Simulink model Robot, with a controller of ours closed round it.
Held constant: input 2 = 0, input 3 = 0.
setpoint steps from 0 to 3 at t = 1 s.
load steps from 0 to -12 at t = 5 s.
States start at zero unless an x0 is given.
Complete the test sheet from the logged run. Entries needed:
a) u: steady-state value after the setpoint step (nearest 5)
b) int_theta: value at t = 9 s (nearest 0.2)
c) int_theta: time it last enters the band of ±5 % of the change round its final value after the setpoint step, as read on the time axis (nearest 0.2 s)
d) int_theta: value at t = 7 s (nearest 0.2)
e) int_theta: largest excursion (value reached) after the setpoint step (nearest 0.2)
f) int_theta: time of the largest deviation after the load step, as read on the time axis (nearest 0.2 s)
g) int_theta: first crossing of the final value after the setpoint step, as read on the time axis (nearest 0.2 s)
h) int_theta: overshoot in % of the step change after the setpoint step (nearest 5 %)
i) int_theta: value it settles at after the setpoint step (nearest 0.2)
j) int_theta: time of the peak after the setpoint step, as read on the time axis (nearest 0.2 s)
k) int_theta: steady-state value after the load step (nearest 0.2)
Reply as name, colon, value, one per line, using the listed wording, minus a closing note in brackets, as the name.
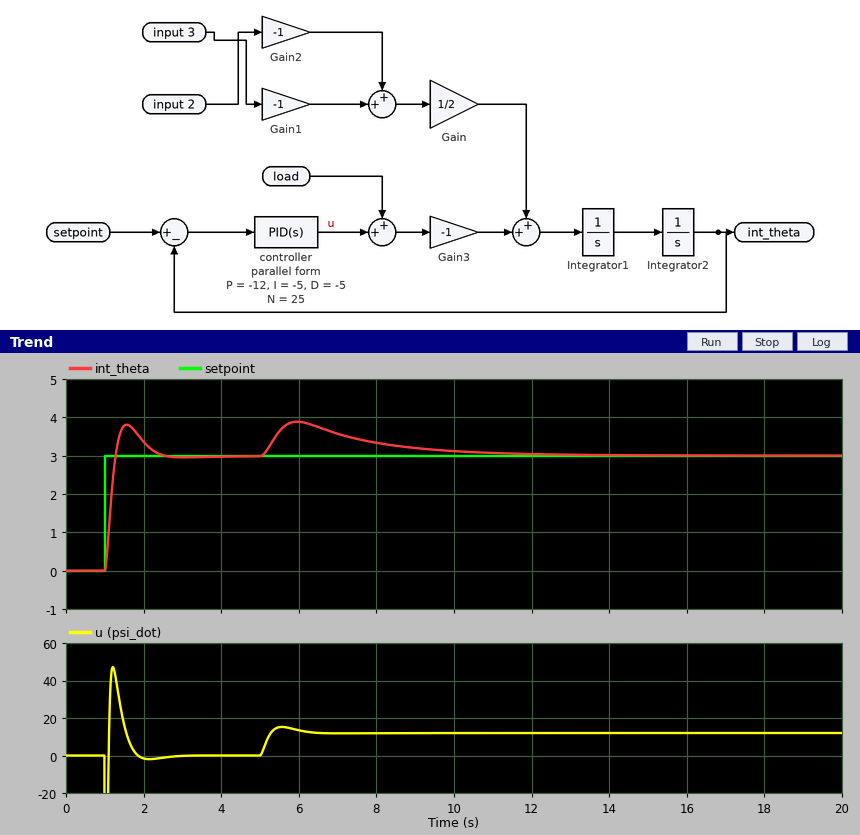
u: steady-state value after the setpoint step: 0
int_theta: value at t = 9 s: 3.2
int_theta: time it last enters the band of ±5 % of the change round its final value after the setpoint step, as read on the time axis: 2.2 s
int_theta: value at t = 7 s: 3.6
int_theta: largest excursion (value reached) after the setpoint step: 3.8
int_theta: time of the largest deviation after the load step, as read on the time axis: 6.0 s
int_theta: first crossing of the final value after the setpoint step, as read on the time axis: 1.2 s
int_theta: overshoot in % of the step change after the setpoint step: 25 %
int_theta: value it settles at after the setpoint step: 3.0
int_theta: time of the peak after the setpoint step, as read on the time axis: 1.6 s
int_theta: steady-state value after the load step: 3.0
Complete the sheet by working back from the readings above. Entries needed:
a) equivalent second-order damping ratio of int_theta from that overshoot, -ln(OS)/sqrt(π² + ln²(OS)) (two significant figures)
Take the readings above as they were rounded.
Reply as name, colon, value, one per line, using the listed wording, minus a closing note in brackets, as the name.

equivalent second-order damping ratio of int_theta from that overshoot, -ln(OS)/sqrt(π² + ln²(OS)): 0.40
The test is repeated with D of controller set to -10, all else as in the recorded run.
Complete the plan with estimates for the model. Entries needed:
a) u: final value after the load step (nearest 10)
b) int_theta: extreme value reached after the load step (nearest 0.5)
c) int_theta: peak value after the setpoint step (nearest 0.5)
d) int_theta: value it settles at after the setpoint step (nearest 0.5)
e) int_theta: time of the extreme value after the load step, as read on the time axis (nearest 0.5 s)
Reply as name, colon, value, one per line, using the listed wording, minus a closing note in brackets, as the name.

u: final value after the load step: 10
int_theta: extreme value reached after the load step: 3.5
int_theta: peak value after the setpoint step: 3.5
int_theta: value it settles at after the setpoint step: 3.0
int_theta: time of the extreme value after the load step, as read on the time axis: 6.5 s
